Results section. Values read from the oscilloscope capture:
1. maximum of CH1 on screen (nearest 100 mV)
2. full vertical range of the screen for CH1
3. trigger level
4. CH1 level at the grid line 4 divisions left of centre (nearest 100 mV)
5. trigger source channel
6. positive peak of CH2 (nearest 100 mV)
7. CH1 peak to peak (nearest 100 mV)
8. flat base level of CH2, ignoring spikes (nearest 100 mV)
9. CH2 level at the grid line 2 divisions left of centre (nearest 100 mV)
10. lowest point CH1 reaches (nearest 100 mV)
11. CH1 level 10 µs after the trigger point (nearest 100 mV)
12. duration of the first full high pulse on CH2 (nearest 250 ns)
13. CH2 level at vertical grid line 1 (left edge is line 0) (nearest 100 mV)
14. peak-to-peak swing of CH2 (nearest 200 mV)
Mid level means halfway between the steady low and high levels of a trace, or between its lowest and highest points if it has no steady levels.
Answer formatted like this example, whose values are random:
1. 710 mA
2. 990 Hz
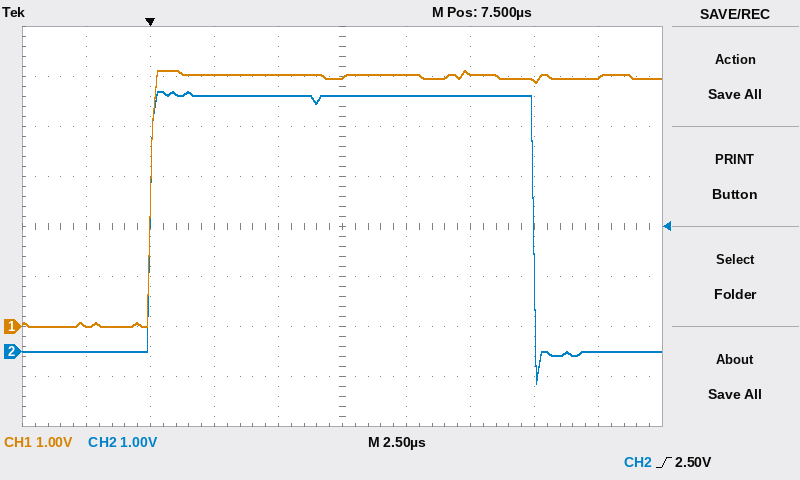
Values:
1. 5.1 V
2. 8 V
3. 2.50 V
4. 0.0 V
5. CH2
6. 5.2 V
7. 5.1 V
8. 0.0 V
9. 5.1 V
10. 0.0 V
11. 5.0 V
12. 15.00 µs
13. 0.0 V
14. 5.8 V
